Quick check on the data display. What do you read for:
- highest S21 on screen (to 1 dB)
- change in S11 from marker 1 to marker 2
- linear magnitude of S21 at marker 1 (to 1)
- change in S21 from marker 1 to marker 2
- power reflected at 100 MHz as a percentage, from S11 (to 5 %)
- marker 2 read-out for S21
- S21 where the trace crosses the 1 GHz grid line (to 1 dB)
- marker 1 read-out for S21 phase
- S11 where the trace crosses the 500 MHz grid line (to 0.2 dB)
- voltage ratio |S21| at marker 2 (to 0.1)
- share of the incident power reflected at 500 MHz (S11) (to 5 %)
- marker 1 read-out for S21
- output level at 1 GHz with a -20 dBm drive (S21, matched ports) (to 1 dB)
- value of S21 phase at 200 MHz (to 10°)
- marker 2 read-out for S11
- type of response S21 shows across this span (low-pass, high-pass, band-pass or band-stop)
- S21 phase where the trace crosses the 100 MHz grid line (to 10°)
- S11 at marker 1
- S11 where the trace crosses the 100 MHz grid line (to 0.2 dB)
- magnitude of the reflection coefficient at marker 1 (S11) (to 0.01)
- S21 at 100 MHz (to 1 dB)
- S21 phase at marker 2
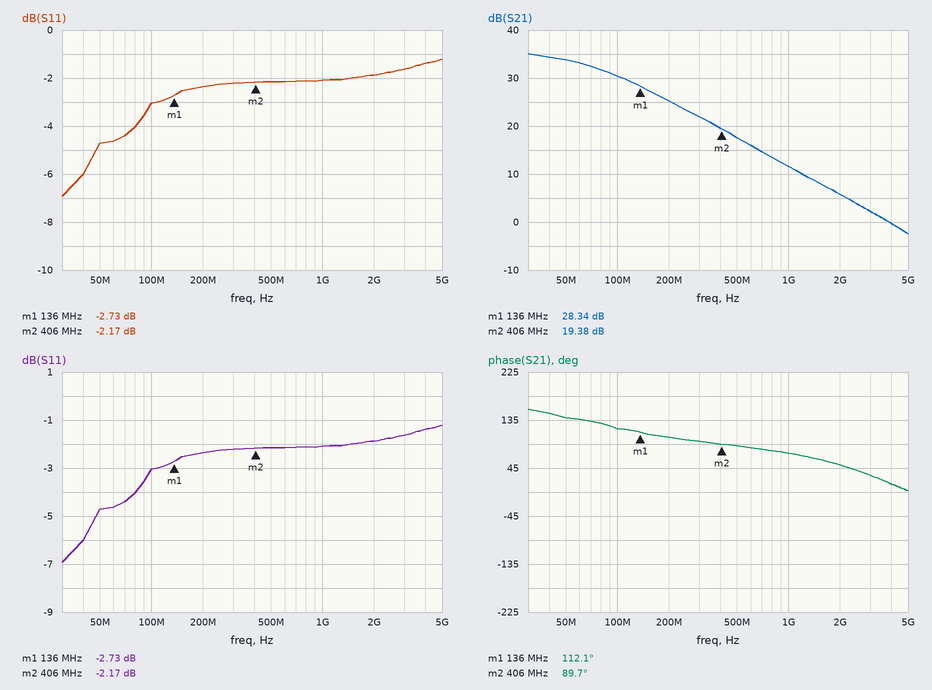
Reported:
35 dB
0.56 dB
26
-8.96 dB
50 %
19.38 dB
12 dB
112.1°
-2.2 dB
9.3
60 %
28.34 dB
-8 dBm
100°
-2.17 dB
low-pass
120°
-2.73 dB
-3.0 dB
0.73
30 dB
89.7°
